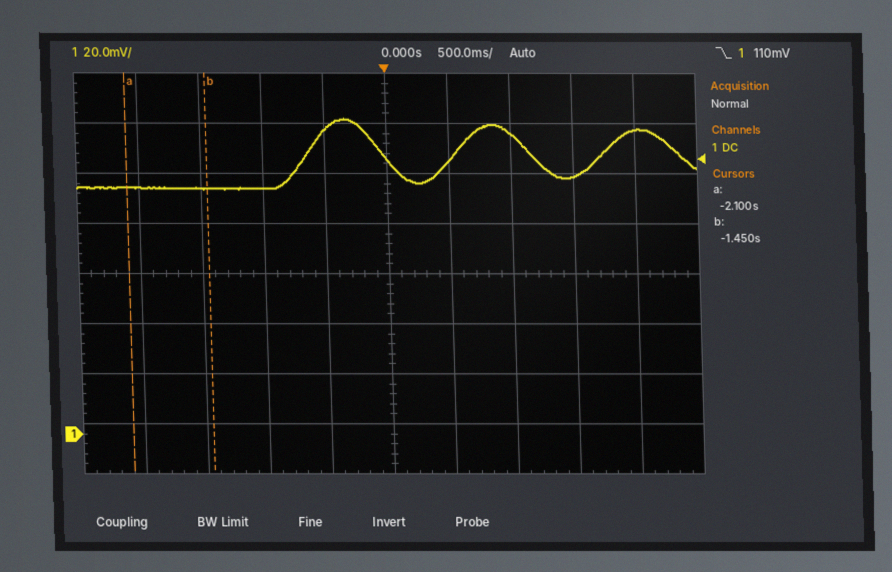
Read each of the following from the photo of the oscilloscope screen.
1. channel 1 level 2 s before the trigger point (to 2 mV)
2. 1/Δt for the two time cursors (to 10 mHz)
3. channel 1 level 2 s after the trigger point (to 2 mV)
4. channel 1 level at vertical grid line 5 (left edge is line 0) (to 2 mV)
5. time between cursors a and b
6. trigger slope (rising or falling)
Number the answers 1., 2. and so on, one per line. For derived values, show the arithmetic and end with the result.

1. 98 mV
2. 1 / 650 ms ≈ 1.54 Hz
3. 122 mV
4. 110 mV
5. -1.45 s − (-2.1 s) = 650 ms
6. falling
